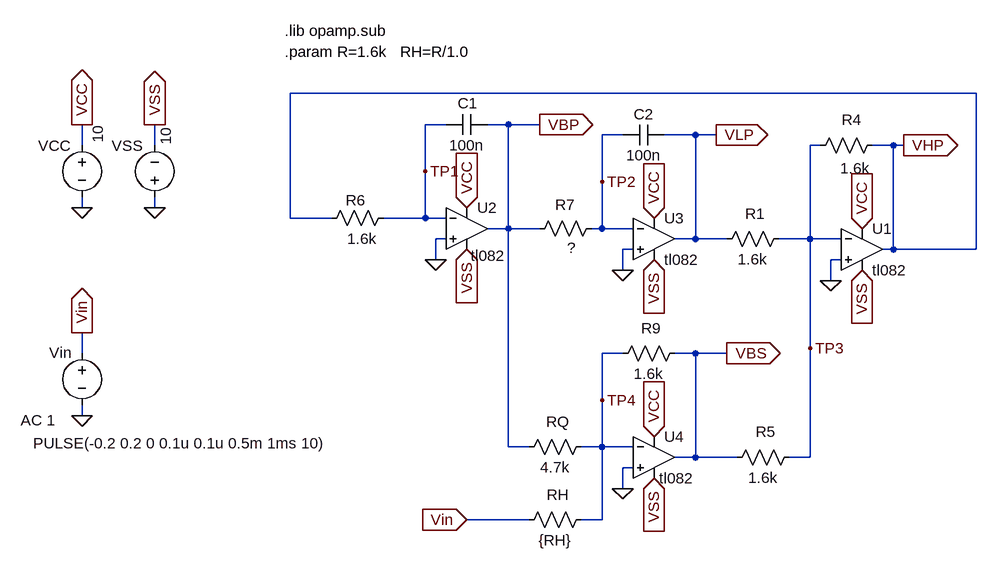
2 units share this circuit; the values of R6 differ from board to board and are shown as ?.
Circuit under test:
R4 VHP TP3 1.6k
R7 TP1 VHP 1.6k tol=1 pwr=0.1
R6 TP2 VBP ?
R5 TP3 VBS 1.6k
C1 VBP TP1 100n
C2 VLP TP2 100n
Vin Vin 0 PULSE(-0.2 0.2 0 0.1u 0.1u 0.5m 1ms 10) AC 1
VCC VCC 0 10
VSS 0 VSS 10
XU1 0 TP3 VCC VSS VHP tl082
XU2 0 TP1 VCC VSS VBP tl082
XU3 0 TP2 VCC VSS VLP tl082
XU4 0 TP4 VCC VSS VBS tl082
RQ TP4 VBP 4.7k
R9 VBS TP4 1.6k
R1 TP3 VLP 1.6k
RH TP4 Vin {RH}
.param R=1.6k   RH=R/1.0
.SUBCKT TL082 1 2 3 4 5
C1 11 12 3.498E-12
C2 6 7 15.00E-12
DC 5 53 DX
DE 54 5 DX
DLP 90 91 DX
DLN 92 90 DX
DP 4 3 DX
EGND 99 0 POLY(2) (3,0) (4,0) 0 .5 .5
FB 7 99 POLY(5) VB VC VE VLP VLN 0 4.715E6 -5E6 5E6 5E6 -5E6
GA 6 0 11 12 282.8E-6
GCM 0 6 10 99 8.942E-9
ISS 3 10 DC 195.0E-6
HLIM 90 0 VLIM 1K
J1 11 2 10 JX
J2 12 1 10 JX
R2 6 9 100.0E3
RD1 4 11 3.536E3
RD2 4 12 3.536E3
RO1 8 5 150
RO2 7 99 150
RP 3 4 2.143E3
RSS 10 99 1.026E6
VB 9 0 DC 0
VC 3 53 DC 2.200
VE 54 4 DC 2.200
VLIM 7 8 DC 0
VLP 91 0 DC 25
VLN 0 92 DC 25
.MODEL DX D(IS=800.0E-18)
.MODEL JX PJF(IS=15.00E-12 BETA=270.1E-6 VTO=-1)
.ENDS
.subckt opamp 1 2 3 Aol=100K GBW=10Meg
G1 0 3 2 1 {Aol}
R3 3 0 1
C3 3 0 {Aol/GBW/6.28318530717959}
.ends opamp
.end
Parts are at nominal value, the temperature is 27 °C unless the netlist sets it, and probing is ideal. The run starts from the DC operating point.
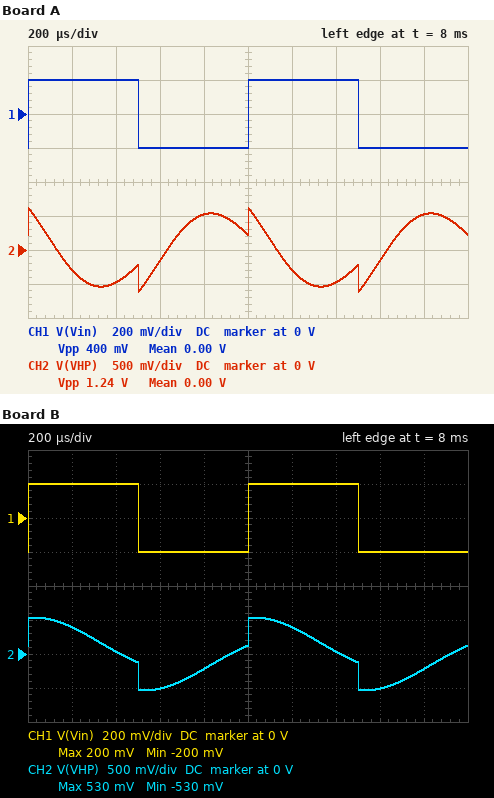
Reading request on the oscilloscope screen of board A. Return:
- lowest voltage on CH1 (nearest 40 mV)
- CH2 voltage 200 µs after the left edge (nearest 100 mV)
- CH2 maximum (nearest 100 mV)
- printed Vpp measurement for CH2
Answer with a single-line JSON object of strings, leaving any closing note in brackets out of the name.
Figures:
{"lowest voltage on CH1": "-200 mV", "CH2 voltage 200 µs after the left edge": "-300 mV", "CH2 maximum": "600 mV", "printed Vpp measurement for CH2": "1.24 V"}
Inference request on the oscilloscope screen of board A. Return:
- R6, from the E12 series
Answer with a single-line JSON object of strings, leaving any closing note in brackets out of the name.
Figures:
{"R6, from the E12 series": "1.2 kΩ"}
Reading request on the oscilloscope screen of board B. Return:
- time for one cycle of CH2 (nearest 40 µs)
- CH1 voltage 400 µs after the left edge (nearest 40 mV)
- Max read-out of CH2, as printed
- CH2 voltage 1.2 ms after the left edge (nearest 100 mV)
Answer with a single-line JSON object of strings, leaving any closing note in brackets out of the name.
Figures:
{"time for one cycle of CH2": "1.00 ms", "CH1 voltage 400 µs after the left edge": "200 mV", "Max read-out of CH2, as printed": "530 mV", "CH2 voltage 1.2 ms after the left edge": "400 mV"}
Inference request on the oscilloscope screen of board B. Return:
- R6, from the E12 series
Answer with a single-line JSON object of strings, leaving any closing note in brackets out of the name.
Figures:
{"R6, from the E12 series": "2.7 kΩ"}
